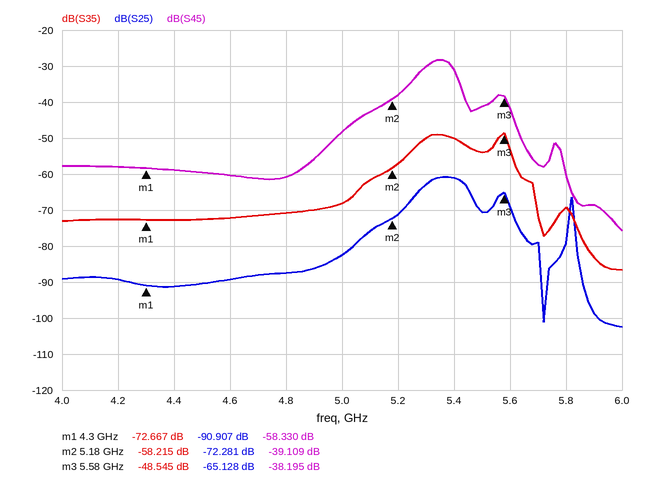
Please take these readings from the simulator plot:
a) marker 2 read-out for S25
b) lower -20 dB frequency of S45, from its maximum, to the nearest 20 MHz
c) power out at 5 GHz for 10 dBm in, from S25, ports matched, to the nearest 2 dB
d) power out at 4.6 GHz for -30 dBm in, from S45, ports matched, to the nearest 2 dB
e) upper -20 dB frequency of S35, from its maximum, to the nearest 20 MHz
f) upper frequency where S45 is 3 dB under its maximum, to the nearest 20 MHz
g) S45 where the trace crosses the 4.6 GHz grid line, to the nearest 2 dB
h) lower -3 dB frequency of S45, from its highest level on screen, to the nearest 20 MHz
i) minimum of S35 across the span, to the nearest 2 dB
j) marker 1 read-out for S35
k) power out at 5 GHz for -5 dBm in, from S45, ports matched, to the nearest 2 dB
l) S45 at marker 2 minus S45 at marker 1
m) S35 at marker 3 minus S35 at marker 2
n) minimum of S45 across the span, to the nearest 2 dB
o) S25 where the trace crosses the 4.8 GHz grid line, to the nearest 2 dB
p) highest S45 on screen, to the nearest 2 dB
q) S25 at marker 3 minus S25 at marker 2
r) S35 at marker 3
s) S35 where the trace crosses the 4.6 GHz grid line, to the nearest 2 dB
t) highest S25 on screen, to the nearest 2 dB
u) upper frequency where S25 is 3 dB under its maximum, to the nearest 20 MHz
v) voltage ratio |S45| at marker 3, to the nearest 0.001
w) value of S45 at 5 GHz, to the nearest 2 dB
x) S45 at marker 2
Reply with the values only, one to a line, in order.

-72.281 dB
5.00 GHz
-72 dBm
-90 dBm
5.70 GHz
5.40 GHz
-60 dB
5.28 GHz
-86 dB
-72.667 dB
-54 dBm
19.221 dB
9.670 dB
-76 dB
-88 dB
-28 dB
7.153 dB
-48.545 dB
-72 dB
-60 dB
5.44 GHz
0.012
-48 dB
-39.109 dB
